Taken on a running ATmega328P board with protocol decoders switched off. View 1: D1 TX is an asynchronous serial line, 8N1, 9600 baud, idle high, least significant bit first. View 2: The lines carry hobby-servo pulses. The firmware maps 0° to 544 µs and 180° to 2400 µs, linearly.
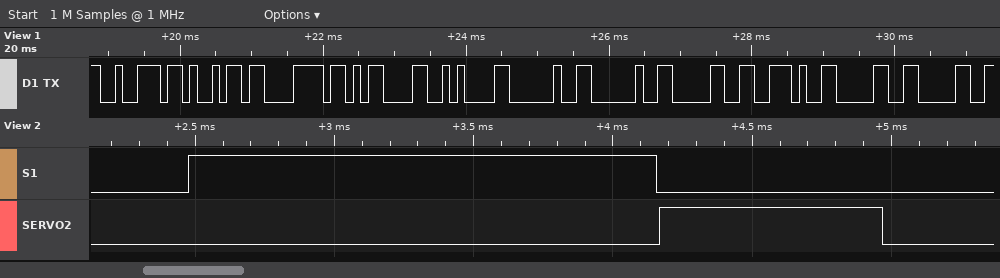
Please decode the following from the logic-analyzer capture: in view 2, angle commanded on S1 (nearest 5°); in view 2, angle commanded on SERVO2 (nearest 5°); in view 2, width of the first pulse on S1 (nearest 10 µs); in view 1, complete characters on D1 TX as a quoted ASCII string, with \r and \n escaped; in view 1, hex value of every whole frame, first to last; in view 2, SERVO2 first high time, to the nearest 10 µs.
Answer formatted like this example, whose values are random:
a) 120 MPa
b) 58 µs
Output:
a) 110°
b) 25°
c) 1680 µs
d) "rix\r\n  0.00"
e) 72 69 78 0D 0A 20 20 30 2E 30 30
f) 800 µs
